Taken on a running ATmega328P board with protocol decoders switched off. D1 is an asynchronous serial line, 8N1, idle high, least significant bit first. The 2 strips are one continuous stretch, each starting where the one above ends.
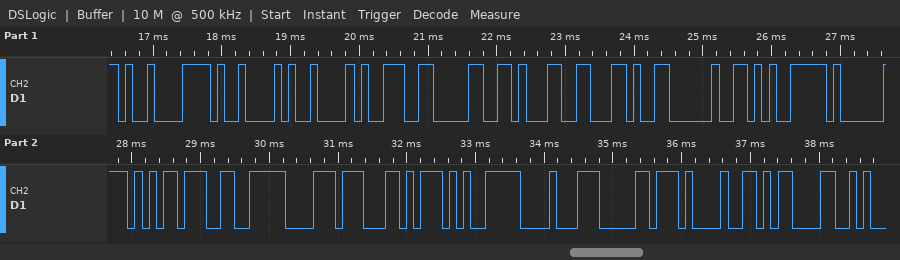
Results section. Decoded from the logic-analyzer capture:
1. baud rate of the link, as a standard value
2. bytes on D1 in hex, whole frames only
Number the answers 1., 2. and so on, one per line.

1. 9600 baud
2. 0x09 0x09 0x09 0x39 0x30 0x31 0x2C 0x20 0xE5 0x81 0xB5 0xE6 0xB8 0xAC 0xE5 0x88 0xB0 0x21 0x0D
